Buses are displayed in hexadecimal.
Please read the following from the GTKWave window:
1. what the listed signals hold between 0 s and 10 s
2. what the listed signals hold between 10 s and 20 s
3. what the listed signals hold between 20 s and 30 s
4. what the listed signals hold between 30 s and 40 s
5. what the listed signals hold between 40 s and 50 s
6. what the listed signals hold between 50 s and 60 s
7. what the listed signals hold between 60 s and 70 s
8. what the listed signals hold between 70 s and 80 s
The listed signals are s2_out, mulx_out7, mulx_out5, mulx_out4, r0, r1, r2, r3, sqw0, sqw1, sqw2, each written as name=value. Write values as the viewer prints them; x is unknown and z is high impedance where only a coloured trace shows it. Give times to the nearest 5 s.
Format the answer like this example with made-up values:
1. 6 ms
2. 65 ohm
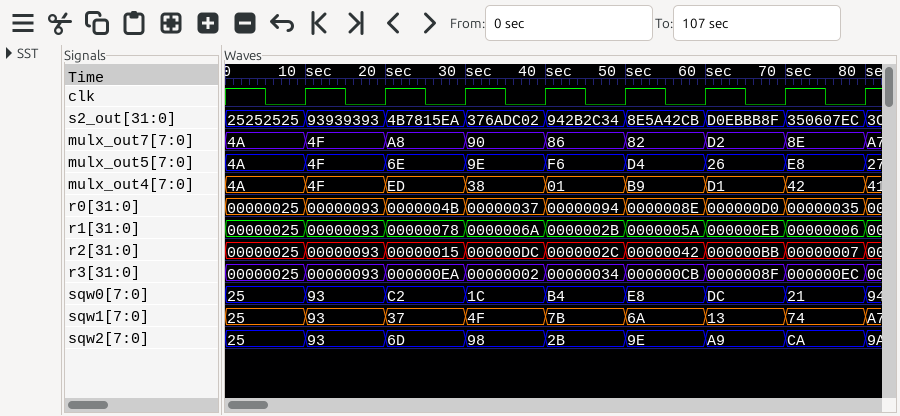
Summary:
1. s2_out=25252525, mulx_out7=4A, mulx_out5=4A, mulx_out4=4A, r0=00000025, r1=00000025, r2=00000025, r3=00000025, sqw0=25, sqw1=25, sqw2=25
2. s2_out=93939393, mulx_out7=4F, mulx_out5=4F, mulx_out4=4F, r0=00000093, r1=00000093, r2=00000093, r3=00000093, sqw0=93, sqw1=93, sqw2=93
3. s2_out=4B7815EA, mulx_out7=A8, mulx_out5=6E, mulx_out4=ED, r0=0000004B, r1=00000078, r2=00000015, r3=000000EA, sqw0=C2, sqw1=37, sqw2=6D
4. s2_out=376ADC02, mulx_out7=90, mulx_out5=9E, mulx_out4=38, r0=00000037, r1=0000006A, r2=000000DC, r3=00000002, sqw0=1C, sqw1=4F, sqw2=98
5. s2_out=942B2C34, mulx_out7=86, mulx_out5=F6, mulx_out4=01, r0=00000094, r1=0000002B, r2=0000002C, r3=00000034, sqw0=B4, sqw1=7B, sqw2=2B
6. s2_out=8E5A42CB, mulx_out7=82, mulx_out5=D4, mulx_out4=B9, r0=0000008E, r1=0000005A, r2=00000042, r3=000000CB, sqw0=E8, sqw1=6A, sqw2=9E
7. s2_out=D0EBBB8F, mulx_out7=D2, mulx_out5=26, mulx_out4=D1, r0=000000D0, r1=000000EB, r2=000000BB, r3=0000008F, sqw0=DC, sqw1=13, sqw2=A9
8. s2_out=350607EC, mulx_out7=8E, mulx_out5=E8, mulx_out4=42, r0=00000035, r1=00000006, r2=00000007, r3=000000EC, sqw0=21, sqw1=74, sqw2=CA
